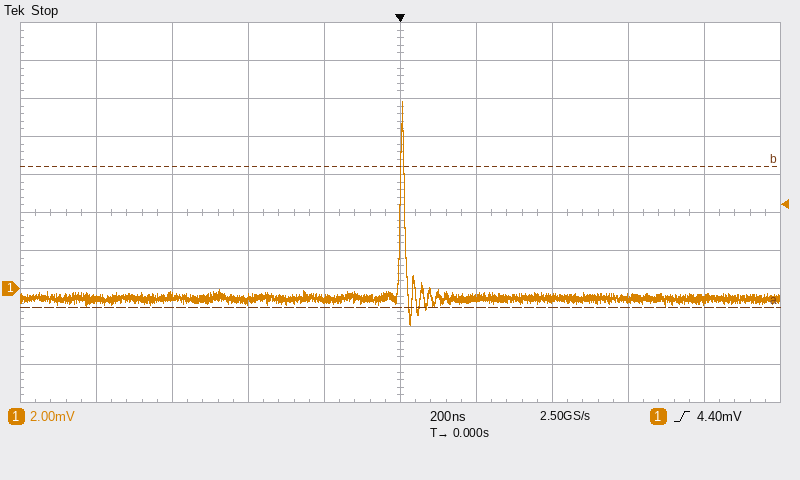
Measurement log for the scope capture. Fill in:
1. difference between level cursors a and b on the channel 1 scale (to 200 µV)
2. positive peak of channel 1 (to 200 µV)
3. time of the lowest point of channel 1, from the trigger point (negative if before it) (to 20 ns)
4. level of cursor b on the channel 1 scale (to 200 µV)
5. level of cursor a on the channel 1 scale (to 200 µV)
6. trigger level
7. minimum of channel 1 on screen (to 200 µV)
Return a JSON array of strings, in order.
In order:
["7.4 mV", "9.8 mV", "+20 ns", "6.4 mV", "-1.0 mV", "4.40 mV", "-1.8 mV"]
